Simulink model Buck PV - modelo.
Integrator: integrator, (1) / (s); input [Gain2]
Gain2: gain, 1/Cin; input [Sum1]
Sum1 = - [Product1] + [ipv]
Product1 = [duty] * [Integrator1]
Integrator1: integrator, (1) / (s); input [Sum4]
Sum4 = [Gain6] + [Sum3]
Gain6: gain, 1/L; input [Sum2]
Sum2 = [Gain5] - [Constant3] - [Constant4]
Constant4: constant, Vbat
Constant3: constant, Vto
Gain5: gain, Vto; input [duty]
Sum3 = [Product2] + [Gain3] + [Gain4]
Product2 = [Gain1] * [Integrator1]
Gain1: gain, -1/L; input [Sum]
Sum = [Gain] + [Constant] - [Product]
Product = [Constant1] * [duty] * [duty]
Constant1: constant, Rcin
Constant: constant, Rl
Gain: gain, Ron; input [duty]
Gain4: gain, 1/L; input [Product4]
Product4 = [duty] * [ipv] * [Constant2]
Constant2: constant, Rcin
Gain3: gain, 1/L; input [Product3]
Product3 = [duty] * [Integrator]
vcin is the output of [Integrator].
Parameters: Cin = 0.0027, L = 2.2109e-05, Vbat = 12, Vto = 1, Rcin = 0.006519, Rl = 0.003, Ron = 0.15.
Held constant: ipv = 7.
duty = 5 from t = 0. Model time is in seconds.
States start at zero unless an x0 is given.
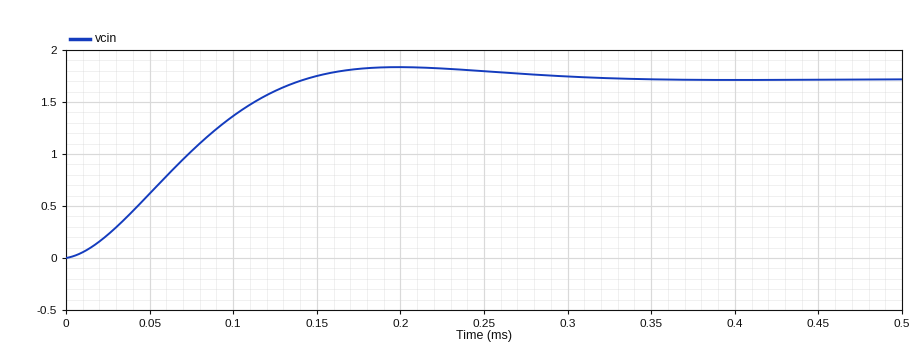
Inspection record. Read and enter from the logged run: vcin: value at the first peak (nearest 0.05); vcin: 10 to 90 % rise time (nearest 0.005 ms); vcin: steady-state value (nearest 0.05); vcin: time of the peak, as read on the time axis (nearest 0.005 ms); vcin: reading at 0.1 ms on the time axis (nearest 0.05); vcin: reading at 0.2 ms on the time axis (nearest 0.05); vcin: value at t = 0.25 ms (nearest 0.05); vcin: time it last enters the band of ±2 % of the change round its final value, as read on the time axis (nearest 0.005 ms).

1.85
0.095 ms
1.70
0.200 ms
1.35
1.85
1.80
0.290 ms
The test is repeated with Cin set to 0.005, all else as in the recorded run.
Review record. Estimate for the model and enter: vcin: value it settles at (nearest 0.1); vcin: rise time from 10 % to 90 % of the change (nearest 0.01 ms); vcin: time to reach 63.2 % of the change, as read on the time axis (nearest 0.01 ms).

1.7
0.19 ms
0.13 ms
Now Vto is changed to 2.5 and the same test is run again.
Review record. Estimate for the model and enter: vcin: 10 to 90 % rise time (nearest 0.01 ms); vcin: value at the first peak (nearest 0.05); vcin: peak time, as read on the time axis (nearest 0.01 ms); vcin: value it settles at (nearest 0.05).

0.09 ms
0.55
0.19 ms
0.50
